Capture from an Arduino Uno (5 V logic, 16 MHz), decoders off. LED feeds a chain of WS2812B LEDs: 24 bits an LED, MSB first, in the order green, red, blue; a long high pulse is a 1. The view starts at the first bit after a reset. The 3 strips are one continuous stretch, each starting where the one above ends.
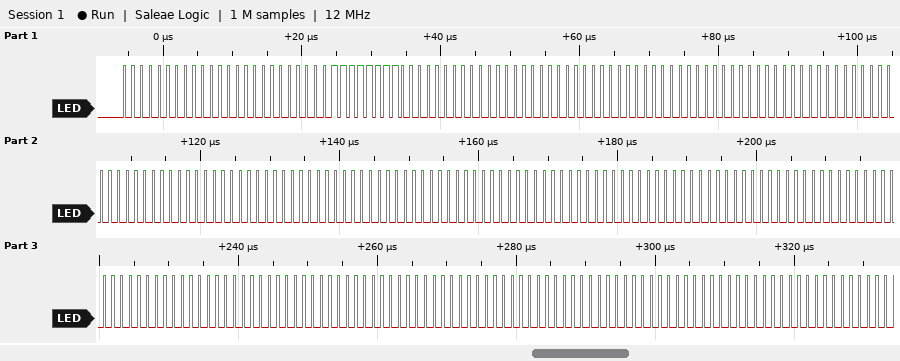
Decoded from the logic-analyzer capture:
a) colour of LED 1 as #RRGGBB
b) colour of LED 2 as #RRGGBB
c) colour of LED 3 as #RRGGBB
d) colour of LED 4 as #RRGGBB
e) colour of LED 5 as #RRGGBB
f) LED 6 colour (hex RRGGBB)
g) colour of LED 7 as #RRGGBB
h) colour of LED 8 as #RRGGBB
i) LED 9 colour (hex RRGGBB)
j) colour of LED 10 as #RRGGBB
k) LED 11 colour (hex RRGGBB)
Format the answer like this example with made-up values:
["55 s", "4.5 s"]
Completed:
["#000000", "#00FF00", "#000000", "#000000", "#000000", "#000000", "#000000", "#000000", "#000000", "#000000", "#000000"]
